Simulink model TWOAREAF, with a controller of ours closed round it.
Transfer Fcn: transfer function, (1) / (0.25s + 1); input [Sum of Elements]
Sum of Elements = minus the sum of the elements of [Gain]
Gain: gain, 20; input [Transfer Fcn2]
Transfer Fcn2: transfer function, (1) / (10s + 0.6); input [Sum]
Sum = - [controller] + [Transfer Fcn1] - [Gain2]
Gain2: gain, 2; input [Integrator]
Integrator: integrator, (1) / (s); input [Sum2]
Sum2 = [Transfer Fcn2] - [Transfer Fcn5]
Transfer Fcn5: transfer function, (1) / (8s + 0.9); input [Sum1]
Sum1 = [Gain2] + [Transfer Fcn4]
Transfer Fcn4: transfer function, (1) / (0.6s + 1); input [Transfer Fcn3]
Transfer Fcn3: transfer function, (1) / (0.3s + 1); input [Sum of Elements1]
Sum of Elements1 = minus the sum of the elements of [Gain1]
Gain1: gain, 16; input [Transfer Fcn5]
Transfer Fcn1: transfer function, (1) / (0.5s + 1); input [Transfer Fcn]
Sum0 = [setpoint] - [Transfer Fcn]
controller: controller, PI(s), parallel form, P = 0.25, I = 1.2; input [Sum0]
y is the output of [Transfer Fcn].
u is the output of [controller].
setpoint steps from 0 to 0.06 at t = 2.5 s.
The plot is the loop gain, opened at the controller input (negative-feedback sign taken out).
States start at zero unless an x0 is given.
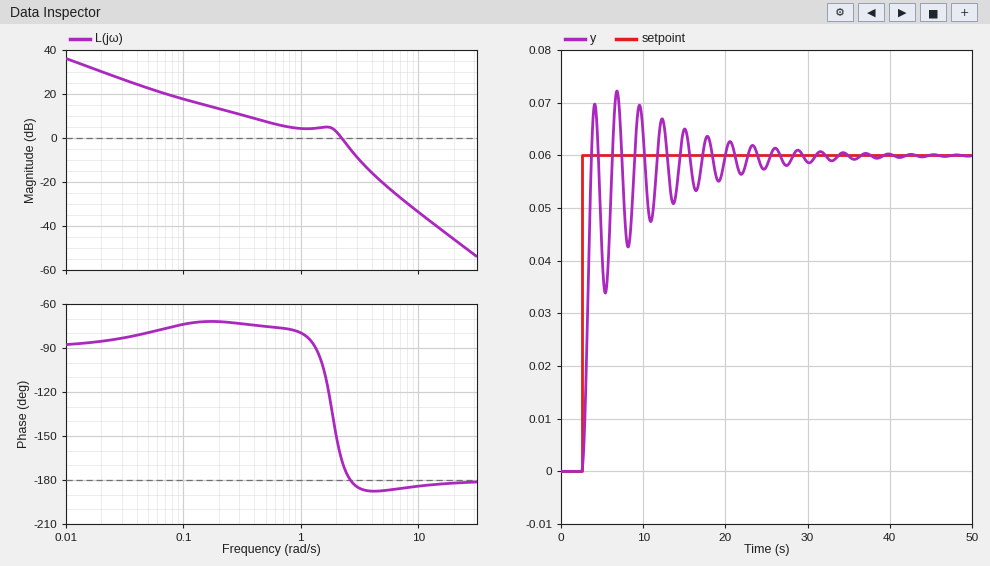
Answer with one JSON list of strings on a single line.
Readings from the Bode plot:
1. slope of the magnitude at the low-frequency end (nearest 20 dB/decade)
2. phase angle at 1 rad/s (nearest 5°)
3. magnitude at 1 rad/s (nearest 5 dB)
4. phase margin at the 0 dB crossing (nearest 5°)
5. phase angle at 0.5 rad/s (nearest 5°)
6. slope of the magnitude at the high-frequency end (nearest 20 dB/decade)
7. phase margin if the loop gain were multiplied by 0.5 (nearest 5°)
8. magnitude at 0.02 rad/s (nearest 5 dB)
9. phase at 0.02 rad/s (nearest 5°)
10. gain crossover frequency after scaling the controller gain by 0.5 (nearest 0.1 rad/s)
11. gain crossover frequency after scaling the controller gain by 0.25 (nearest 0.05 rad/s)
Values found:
["-20 dB/decade", "-80°", "5 dB", "15°", "-75°", "-40 dB/decade", "105°", "30 dB", "-85°", "0.6 rad/s", "0.25 rad/s"]
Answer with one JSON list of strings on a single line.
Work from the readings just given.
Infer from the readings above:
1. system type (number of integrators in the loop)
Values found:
["1"]
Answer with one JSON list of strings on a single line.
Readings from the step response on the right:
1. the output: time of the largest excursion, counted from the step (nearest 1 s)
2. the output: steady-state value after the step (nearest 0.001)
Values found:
["4 s", "0.060"]
